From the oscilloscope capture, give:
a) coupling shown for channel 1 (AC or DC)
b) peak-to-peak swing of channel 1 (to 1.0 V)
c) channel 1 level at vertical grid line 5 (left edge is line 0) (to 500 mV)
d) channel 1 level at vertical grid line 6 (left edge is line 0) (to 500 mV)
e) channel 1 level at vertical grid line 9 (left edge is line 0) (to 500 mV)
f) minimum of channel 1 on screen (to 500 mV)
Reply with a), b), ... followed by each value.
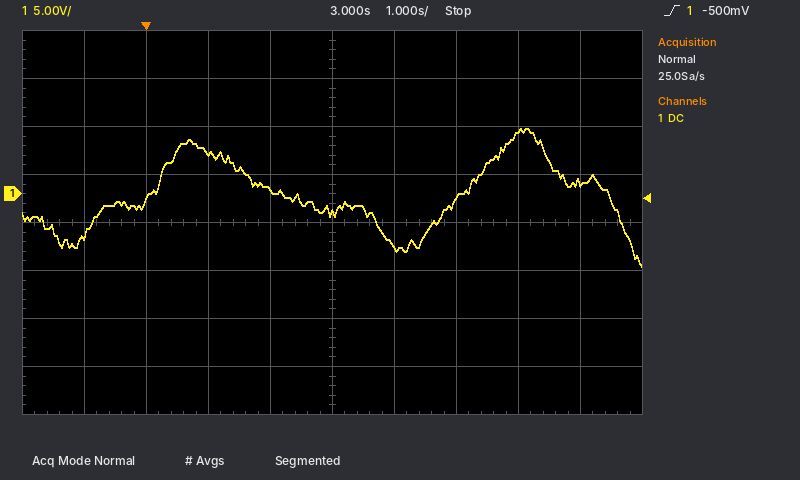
a) DC
b) 14.0 V
c) -2.0 V
d) -5.5 V
e) 1.0 V
f) -7.5 V
